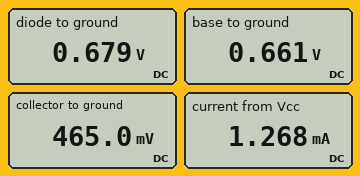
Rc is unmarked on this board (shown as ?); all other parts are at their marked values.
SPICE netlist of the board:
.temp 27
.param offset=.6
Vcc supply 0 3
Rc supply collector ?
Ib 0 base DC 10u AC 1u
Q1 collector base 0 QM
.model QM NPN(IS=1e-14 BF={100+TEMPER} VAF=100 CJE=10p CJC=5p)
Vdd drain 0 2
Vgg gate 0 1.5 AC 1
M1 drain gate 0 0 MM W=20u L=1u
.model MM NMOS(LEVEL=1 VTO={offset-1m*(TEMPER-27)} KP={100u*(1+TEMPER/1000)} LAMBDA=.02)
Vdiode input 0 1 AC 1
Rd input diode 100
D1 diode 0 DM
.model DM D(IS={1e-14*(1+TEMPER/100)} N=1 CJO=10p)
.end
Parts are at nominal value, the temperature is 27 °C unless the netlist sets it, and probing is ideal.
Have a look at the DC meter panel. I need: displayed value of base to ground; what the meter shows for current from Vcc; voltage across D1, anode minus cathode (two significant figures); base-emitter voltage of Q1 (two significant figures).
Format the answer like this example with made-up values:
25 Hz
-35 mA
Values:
0.661 V
1.268 mA
680 mV
660 mV
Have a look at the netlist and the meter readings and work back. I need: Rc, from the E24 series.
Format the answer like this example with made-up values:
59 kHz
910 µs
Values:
2 kΩ
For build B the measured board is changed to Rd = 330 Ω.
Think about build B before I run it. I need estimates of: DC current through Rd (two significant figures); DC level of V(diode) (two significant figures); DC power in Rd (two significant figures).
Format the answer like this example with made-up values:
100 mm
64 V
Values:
1.1 mA
650 mV
370 µW
